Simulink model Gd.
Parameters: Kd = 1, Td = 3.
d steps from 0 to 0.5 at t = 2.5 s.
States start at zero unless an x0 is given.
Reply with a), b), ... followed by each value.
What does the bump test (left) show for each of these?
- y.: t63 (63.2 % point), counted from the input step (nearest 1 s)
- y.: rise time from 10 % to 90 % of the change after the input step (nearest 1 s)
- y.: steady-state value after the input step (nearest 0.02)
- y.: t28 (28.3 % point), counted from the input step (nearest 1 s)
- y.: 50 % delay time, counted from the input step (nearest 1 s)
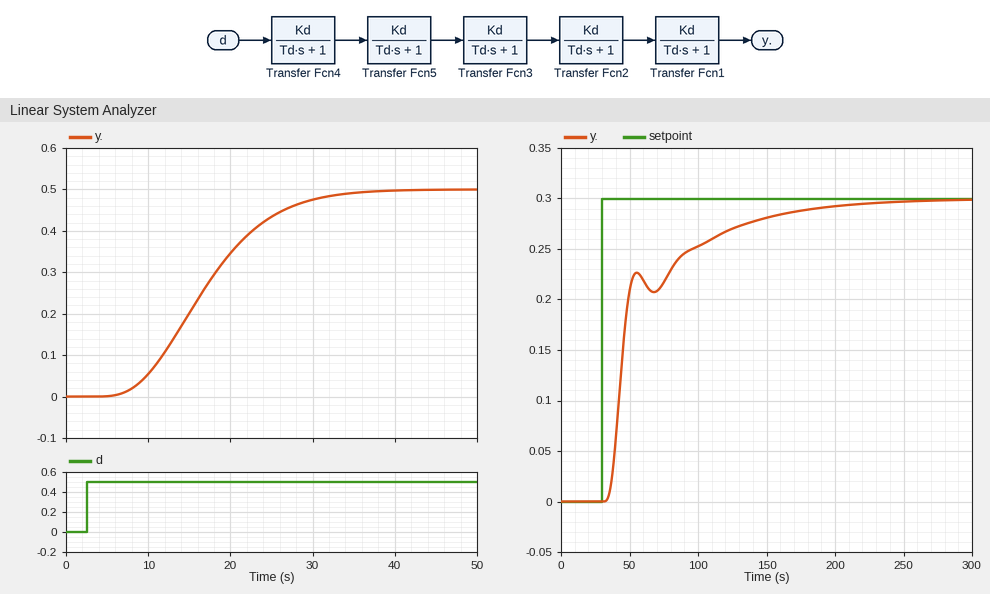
a) 16 s
b) 17 s
c) 0.50
d) 11 s
e) 14 s
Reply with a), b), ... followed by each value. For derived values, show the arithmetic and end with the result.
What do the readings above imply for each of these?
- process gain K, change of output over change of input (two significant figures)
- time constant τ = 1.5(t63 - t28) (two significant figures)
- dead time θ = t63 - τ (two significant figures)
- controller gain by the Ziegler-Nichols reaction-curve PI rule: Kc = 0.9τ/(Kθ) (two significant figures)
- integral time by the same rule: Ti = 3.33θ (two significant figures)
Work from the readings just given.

a) (0.5 - 0) / 0.5 = 1.0
b) 1.5 × (16 - 11) = 7.5 s
c) 16 - 7.5 = 8.5 s
d) 0.9 × 7.5 / (1 × 8.5) = 0.79
e) 3.33 × 8.5 = 28 s
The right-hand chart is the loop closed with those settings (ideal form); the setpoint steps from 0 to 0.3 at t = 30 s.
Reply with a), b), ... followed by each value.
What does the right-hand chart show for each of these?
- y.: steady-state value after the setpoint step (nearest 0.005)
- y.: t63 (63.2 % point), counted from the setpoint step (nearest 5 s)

a) 0.300
b) 20 s
